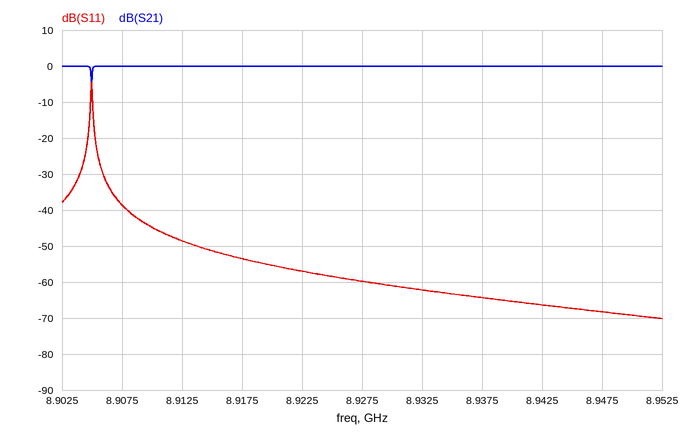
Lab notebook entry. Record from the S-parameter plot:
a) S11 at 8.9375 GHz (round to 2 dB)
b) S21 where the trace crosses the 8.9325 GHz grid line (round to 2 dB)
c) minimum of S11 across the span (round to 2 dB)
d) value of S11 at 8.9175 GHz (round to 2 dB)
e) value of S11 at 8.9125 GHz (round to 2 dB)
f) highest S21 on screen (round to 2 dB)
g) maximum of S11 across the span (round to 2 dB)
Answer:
-64 dB
0 dB
-70 dB
-54 dB
-48 dB
0 dB
-4 dB
